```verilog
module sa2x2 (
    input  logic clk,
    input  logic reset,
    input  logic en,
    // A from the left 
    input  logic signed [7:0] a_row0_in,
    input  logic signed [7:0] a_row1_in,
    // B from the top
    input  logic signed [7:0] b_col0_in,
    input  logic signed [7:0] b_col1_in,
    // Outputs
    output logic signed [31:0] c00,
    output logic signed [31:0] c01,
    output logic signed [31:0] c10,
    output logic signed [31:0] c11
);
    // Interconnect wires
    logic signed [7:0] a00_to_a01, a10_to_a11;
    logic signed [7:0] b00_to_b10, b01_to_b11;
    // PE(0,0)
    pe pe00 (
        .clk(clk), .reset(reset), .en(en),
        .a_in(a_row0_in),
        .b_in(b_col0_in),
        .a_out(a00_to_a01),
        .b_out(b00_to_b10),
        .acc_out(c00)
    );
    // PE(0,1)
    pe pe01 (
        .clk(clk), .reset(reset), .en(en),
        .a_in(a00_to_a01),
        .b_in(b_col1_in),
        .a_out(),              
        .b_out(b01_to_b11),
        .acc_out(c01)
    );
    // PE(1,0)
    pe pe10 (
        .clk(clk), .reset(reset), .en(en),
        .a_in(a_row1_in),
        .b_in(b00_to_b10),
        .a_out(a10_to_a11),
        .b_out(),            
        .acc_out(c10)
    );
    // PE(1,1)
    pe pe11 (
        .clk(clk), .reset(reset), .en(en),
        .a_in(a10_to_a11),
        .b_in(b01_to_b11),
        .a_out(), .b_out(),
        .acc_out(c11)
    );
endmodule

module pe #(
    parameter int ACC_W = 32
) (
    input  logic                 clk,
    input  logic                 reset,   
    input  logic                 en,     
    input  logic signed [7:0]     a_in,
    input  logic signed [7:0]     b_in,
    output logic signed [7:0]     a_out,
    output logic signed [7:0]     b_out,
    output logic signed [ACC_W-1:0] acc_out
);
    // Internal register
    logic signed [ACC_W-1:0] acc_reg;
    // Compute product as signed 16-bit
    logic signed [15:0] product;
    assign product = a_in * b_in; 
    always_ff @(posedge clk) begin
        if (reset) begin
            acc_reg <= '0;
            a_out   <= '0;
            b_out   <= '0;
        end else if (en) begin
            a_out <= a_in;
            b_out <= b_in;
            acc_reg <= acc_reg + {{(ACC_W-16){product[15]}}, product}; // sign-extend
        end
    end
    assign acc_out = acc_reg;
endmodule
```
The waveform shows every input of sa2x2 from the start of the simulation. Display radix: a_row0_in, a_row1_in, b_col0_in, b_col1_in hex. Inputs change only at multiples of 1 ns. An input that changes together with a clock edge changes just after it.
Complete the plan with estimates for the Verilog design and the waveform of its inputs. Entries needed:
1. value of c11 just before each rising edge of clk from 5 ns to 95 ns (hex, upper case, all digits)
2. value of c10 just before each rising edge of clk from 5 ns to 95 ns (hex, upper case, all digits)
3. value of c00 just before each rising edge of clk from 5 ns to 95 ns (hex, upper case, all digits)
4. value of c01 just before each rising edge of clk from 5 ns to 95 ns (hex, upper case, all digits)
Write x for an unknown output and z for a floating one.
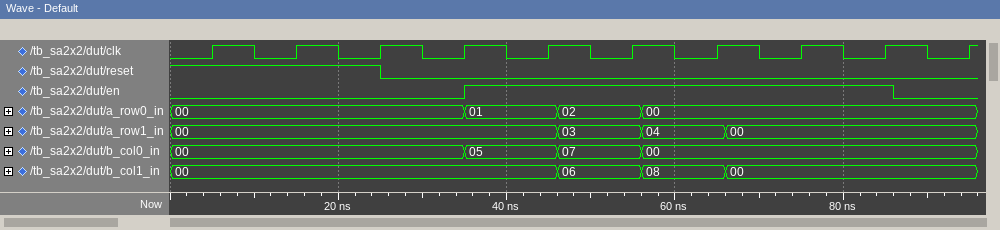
x, 00000000, 00000000, 00000000, 00000000, 00000000, 00000000, 00000012, 00000032, 00000032
x, 00000000, 00000000, 00000000, 00000000, 00000000, 0000000F, 0000002B, 0000002B, 0000002B
x, 00000000, 00000000, 00000000, 00000000, 00000005, 00000013, 00000013, 00000013, 00000013
x, 00000000, 00000000, 00000000, 00000000, 00000000, 00000006, 00000016, 00000016, 00000016
